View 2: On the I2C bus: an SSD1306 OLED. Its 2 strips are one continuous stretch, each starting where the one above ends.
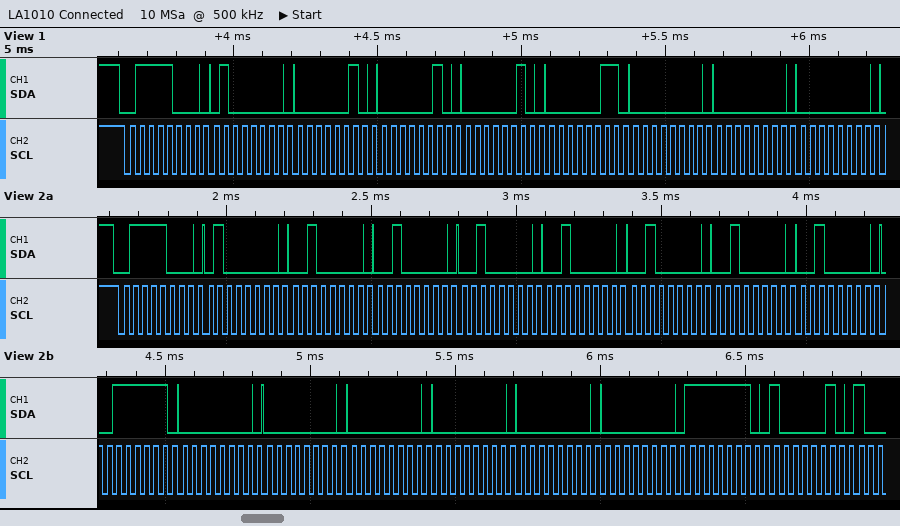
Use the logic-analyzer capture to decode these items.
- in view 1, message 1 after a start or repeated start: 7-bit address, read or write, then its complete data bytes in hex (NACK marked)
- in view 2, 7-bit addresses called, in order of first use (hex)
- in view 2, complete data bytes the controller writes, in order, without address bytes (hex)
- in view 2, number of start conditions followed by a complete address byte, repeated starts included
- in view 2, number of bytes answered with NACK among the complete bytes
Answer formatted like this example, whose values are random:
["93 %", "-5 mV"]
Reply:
["0x3C write: 40 02 02 02 03 00 00 00", "0x3C", "40 20 20 20 20 20 20 20 3F 00 00 00 00 00 00 FE 82", "1", "0"]
